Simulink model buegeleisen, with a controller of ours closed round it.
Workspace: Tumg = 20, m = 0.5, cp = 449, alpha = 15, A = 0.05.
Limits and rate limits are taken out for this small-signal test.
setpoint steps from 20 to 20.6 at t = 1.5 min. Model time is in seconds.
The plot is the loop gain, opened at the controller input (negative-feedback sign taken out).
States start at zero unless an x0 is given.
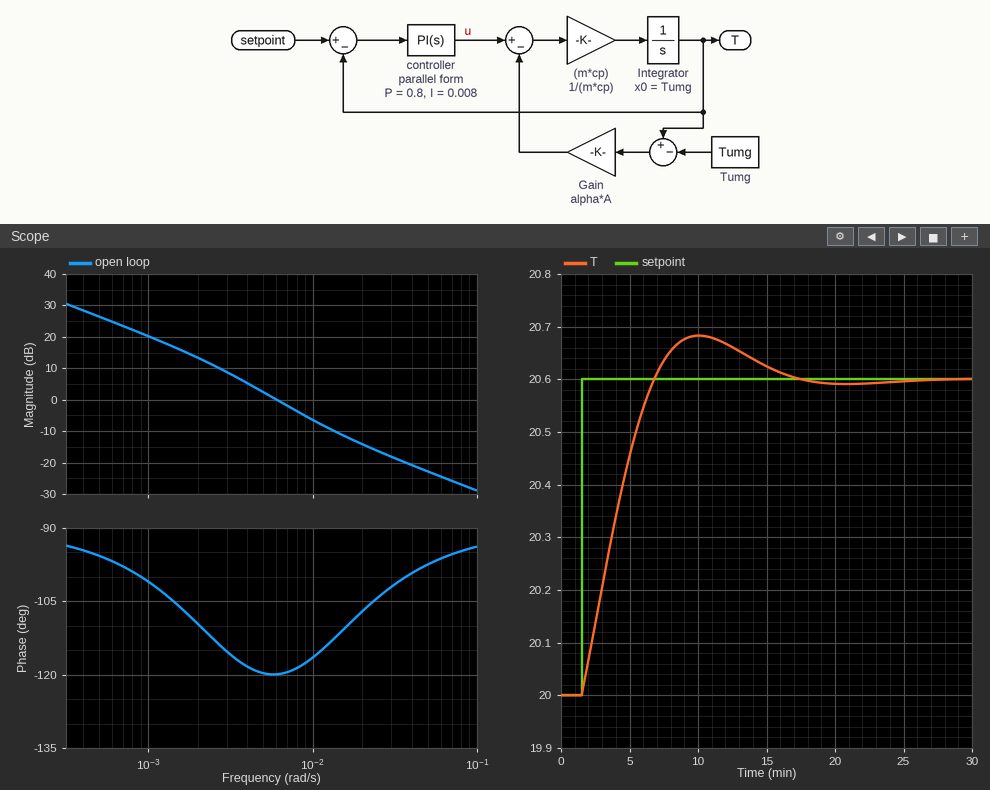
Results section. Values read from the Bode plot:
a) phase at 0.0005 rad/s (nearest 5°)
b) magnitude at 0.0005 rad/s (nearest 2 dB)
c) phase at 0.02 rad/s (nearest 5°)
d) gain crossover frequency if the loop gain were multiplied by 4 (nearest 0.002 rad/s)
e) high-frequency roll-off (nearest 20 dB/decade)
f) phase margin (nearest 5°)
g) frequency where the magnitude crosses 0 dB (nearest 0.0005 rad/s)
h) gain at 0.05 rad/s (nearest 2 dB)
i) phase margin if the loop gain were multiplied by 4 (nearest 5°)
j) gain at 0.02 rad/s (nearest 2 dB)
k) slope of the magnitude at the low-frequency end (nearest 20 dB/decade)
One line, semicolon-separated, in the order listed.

-95°; 26 dB; -105°; 0.016 rad/s; -20 dB/decade; 60°; 0.0060 rad/s; -22 dB; 70°; -14 dB; -20 dB/decade
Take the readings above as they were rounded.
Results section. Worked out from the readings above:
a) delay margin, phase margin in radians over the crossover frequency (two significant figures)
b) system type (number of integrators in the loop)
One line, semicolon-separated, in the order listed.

170 s; 1
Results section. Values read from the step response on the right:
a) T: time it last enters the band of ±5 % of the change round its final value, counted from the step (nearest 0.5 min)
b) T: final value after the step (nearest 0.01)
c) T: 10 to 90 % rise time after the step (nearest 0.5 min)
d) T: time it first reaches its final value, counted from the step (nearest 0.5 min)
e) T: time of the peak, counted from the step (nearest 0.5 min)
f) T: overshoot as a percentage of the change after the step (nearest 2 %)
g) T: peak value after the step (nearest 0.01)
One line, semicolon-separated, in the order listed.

13.0 min; 20.60; 4.0 min; 5.5 min; 8.5 min; 14 %; 20.68
